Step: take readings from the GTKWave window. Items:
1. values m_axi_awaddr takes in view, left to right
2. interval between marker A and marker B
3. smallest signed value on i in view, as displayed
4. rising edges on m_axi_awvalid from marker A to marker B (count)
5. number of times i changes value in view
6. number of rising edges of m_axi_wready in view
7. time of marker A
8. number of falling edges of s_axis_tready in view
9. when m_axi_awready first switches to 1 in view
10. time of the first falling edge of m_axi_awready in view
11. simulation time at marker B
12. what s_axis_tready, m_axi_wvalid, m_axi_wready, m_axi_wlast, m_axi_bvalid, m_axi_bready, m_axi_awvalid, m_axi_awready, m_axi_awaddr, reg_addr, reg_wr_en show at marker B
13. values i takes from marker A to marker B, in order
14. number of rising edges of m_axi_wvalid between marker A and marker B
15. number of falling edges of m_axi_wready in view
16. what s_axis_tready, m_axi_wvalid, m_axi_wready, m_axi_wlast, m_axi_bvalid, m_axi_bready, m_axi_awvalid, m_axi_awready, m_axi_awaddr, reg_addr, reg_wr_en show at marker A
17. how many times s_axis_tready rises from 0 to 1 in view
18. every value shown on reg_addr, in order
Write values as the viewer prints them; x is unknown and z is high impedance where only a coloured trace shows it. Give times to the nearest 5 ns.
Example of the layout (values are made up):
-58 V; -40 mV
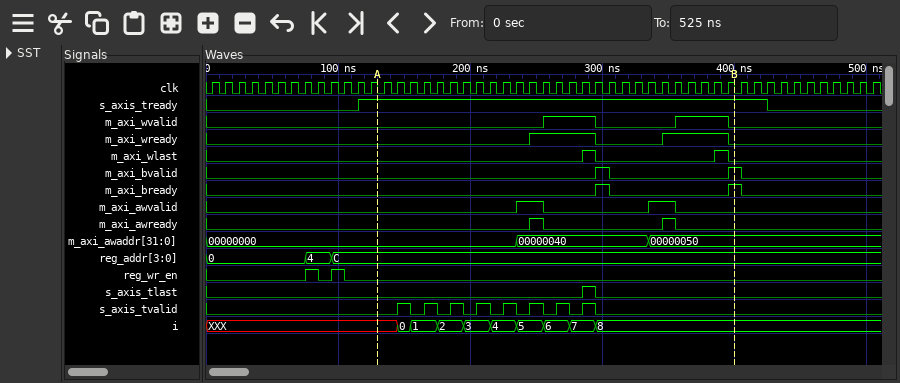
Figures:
00000000, 00000040, 00000050; 270 ns; 0; 2; 9; 2; 130 ns; 1; 245 ns; 255 ns; 400 ns; s_axis_tready=1, m_axi_wvalid=0, m_axi_wready=0, m_axi_wlast=0, m_axi_bvalid=1, m_axi_bready=1, m_axi_awvalid=0, m_axi_awready=0, m_axi_awaddr=00000050, reg_addr=C, reg_wr_en=0; XXX, 0, 1, 2, 3, 4, 5, 6, 7, 8; 2; 2; s_axis_tready=1, m_axi_wvalid=0, m_axi_wready=0, m_axi_wlast=0, m_axi_bvalid=0, m_axi_bready=0, m_axi_awvalid=0, m_axi_awready=0, m_axi_awaddr=00000000, reg_addr=C, reg_wr_en=0; 1; 0, 4, C
